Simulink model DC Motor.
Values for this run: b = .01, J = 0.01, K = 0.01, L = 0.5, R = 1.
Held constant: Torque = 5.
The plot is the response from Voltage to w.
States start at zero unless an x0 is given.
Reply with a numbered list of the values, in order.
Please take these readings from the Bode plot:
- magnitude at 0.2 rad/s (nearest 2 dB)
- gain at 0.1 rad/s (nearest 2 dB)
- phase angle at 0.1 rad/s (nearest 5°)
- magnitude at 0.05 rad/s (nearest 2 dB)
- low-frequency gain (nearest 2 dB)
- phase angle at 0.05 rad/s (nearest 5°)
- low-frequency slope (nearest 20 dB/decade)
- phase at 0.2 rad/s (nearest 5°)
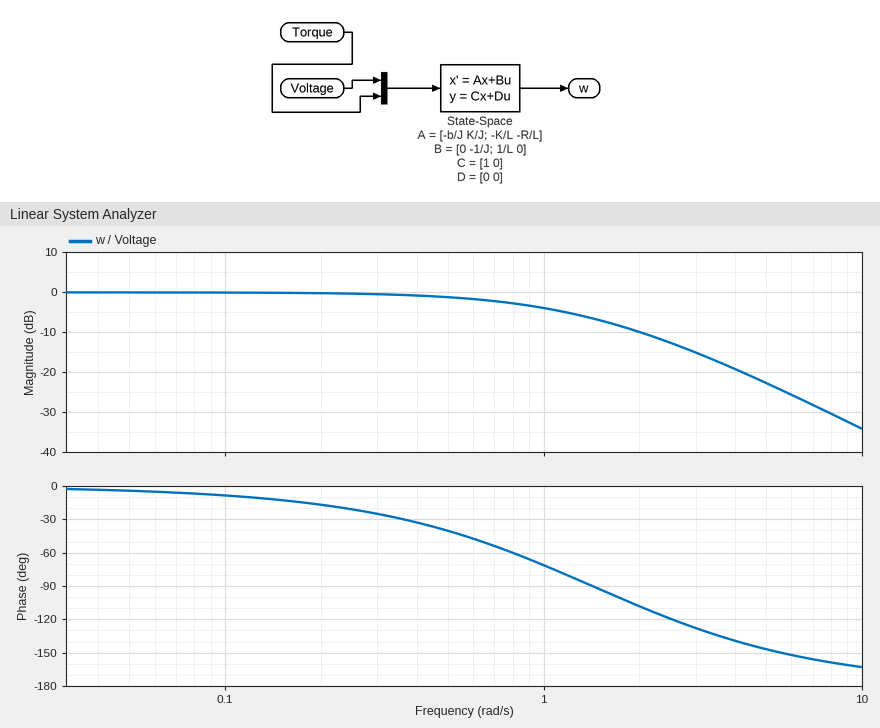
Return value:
1. 0 dB
2. 0 dB
3. -10°
4. 0 dB
5. 0 dB
6. -5°
7. 0 dB/decade
8. -15°
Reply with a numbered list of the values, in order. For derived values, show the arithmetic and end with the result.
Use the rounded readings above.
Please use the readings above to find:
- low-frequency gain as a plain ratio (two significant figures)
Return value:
1. 10^(0 / 20) = 1.0
